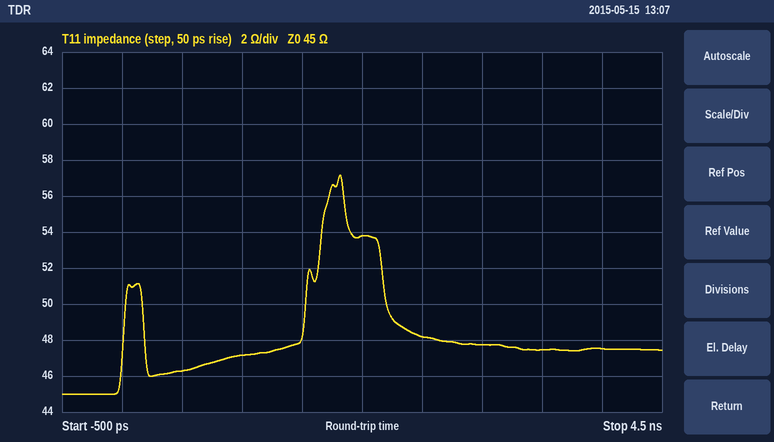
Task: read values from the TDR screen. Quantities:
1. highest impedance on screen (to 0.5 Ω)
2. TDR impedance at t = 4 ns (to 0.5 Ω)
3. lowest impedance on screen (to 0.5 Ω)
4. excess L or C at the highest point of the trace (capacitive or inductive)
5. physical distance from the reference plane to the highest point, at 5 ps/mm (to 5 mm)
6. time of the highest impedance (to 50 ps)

57.0 Ω
47.5 Ω
45.0 Ω
inductive
180 mm
1.80 ns
